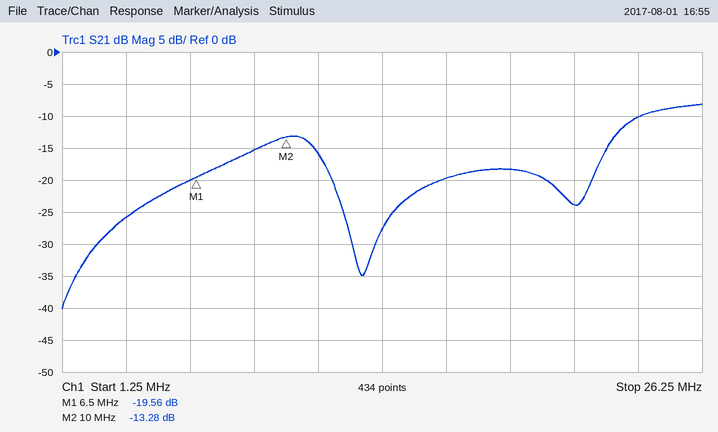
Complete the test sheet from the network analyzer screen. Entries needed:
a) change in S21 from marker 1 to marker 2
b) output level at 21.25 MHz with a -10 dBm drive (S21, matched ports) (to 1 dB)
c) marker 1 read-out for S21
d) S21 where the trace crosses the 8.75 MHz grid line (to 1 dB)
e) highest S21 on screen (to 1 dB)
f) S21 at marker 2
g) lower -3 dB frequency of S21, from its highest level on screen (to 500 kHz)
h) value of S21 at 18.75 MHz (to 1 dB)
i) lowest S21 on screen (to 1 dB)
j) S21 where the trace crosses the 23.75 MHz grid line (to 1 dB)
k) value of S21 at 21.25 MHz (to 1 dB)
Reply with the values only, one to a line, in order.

6.28 dB
-34 dBm
-19.56 dB
-15 dB
-8 dB
-13.28 dB
23.5 MHz
-18 dB
-40 dB
-10 dB
-24 dB
